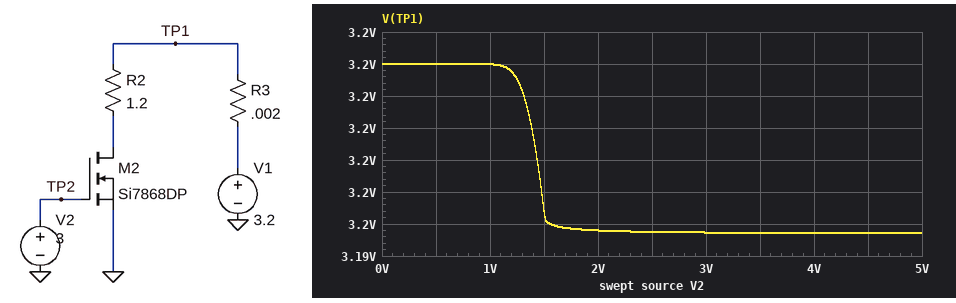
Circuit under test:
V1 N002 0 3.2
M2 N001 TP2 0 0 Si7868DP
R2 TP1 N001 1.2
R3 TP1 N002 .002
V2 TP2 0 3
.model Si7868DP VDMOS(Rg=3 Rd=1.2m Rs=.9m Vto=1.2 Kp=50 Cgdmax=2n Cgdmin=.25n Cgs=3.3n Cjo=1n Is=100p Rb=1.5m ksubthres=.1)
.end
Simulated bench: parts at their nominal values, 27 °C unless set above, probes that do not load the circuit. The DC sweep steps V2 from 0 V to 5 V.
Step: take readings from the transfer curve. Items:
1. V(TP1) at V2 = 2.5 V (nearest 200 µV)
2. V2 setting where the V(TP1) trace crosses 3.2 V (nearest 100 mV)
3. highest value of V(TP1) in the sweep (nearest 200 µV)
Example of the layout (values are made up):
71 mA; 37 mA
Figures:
3.1948 V; 1.4 V; 3.2000 V
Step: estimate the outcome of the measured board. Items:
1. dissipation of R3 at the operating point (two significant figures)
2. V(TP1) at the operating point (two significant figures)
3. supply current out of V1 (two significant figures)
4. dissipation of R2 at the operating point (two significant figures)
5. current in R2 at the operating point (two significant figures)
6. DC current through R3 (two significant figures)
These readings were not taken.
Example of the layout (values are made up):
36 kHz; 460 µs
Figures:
14 mW; 3.2 V; 2.6 A; 8.3 W; 2.6 A; 2.6 A
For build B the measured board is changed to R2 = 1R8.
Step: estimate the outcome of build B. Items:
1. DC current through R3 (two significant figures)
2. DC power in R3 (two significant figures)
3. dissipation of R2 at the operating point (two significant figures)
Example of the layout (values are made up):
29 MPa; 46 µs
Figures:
1.8 A; 6.2 mW; 5.6 W
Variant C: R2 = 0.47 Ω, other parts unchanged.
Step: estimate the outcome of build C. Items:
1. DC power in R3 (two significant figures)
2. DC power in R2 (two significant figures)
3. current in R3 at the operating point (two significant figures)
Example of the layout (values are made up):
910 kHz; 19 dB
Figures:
87 mW; 20 W; 6.6 A
